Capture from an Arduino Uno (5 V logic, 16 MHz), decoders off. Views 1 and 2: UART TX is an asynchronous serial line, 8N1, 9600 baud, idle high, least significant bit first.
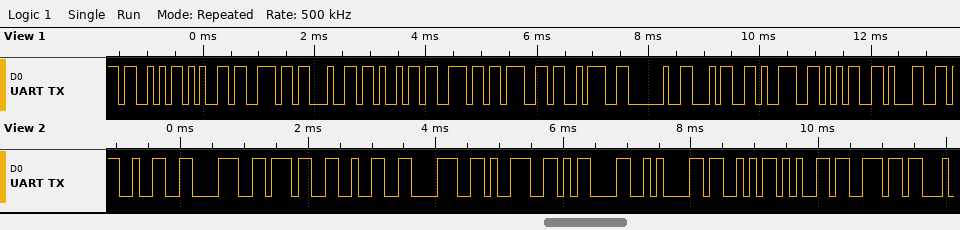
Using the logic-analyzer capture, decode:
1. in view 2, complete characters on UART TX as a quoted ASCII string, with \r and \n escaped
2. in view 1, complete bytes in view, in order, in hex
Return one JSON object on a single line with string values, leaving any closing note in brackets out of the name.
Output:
{"in view 2, complete characters on UART TX as a quoted ASCII string, with \\r and \\n escaped": "\"287289\\r\\nSen\"", "in view 1, complete bytes in view, in order, in hex": "53 65 6E 64 69 6E 67 3A 20 34 39 35 31"}
